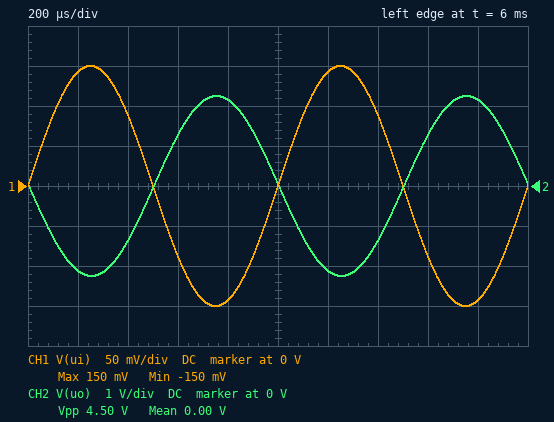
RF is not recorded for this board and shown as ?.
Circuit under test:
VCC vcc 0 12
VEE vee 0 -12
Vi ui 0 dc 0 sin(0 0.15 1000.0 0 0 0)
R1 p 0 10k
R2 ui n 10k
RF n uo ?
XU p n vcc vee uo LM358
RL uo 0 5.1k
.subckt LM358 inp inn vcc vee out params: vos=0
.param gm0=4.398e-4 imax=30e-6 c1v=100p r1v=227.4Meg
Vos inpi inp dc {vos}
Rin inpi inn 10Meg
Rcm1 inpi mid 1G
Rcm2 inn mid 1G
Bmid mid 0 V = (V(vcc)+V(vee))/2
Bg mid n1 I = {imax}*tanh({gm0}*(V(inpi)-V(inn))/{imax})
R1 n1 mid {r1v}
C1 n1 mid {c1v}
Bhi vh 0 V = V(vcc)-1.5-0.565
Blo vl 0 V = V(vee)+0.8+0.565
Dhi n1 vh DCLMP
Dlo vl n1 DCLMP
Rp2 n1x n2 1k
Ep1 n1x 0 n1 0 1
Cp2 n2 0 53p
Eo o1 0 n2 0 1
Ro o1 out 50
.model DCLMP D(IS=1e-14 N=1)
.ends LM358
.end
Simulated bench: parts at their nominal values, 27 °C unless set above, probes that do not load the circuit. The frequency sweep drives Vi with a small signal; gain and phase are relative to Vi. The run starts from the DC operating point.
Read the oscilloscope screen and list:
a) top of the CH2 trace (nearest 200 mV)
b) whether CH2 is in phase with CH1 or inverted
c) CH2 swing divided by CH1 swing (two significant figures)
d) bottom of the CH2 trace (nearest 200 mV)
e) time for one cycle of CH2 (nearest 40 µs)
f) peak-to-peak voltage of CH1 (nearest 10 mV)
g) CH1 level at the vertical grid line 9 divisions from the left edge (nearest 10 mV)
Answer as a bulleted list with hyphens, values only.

- 2.2 V
- inverted
- 15
- -2.2 V
- 1.00 ms
- 300 mV
- -140 mV
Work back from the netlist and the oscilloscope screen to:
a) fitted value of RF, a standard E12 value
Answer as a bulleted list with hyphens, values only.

- 150 kΩ
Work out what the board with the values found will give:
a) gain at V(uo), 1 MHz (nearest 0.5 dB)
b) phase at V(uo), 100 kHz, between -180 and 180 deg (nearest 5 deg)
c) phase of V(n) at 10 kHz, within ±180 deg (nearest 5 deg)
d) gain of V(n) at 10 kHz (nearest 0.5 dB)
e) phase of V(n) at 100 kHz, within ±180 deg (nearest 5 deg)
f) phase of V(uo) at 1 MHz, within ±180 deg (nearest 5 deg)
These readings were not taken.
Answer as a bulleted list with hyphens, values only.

- -4.0 dB
- 110 deg
- 75 deg
- -13.5 dB
- 25 deg
- 75 deg
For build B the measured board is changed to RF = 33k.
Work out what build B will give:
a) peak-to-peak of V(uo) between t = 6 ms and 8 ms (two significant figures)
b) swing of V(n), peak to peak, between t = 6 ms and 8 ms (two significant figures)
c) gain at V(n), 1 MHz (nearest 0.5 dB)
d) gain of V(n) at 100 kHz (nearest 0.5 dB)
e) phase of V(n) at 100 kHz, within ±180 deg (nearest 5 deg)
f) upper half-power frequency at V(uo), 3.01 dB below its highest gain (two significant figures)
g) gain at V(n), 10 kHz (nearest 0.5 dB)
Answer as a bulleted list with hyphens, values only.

- 990 mV
- 1.4 mV
- -2.0 dB
- -7.5 dB
- 60 deg
- 170 kHz
- -26.5 dB
